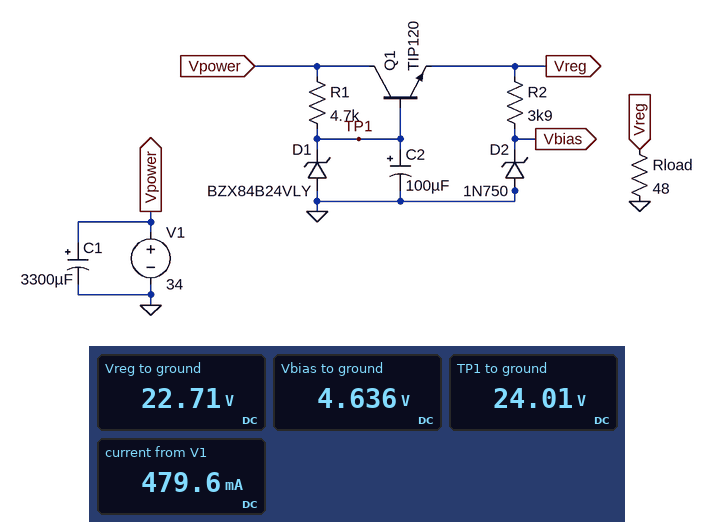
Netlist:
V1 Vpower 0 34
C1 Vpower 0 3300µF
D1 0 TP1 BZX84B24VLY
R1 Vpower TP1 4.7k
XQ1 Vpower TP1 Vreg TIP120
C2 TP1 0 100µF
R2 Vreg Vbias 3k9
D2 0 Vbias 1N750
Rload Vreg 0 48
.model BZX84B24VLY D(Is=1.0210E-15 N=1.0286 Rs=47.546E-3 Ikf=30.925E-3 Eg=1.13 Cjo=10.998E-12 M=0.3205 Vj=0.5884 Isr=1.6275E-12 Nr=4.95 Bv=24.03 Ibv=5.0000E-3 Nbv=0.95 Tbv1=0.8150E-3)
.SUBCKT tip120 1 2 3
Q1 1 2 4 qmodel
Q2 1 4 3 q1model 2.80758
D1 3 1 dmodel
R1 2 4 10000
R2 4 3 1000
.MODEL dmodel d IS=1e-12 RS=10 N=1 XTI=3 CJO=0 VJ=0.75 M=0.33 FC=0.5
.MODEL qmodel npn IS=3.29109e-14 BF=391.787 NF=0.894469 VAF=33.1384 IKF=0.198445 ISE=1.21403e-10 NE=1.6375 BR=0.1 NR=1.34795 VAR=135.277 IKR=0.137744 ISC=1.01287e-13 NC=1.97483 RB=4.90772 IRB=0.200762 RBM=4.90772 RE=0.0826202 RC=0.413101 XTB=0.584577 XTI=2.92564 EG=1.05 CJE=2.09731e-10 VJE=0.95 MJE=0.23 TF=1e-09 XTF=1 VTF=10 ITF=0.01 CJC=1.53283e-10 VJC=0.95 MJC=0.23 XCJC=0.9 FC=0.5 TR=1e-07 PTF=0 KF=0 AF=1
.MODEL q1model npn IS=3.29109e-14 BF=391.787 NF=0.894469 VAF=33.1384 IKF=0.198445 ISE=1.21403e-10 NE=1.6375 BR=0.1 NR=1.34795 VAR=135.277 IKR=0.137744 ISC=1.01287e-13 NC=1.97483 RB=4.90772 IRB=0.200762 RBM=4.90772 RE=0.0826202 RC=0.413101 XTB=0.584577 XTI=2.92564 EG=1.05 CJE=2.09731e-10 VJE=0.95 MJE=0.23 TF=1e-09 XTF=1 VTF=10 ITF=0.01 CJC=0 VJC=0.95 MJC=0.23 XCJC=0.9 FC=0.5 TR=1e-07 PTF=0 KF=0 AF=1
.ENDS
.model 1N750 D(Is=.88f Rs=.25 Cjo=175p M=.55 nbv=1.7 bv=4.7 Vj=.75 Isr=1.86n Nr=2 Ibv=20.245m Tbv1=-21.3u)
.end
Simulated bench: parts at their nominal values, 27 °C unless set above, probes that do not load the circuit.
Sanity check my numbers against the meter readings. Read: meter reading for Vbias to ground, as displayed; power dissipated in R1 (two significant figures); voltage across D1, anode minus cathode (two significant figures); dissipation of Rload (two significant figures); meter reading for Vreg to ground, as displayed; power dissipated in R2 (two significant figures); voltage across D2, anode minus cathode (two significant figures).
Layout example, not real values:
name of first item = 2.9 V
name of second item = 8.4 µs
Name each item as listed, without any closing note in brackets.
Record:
meter reading for Vbias to ground, as displayed = 4.636 V
power dissipated in R1 = 21 mW
voltage across D1, anode minus cathode = -24 V
dissipation of Rload = 11 W
meter reading for Vreg to ground, as displayed = 22.71 V
power dissipated in R2 = 84 mW
voltage across D2, anode minus cathode = -4.6 V
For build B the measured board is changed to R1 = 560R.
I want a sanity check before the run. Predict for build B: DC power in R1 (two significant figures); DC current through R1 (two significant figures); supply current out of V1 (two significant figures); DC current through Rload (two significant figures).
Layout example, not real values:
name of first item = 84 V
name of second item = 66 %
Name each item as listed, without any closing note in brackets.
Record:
DC power in R1 = 180 mW
DC current through R1 = 18 mA
supply current out of V1 = 500 mA
DC current through Rload = 470 mA
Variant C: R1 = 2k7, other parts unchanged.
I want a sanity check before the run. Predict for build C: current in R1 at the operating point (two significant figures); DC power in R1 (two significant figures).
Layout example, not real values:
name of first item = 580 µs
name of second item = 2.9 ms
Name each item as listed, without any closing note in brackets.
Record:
current in R1 at the operating point = 3.7 mA
DC power in R1 = 37 mW
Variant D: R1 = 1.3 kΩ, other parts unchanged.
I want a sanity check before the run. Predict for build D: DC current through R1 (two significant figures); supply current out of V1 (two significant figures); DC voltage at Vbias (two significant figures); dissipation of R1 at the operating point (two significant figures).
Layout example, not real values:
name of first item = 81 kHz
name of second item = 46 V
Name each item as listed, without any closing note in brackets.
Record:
DC current through R1 = 7.7 mA
supply current out of V1 = 490 mA
DC voltage at Vbias = 4.6 V
dissipation of R1 at the operating point = 76 mW
